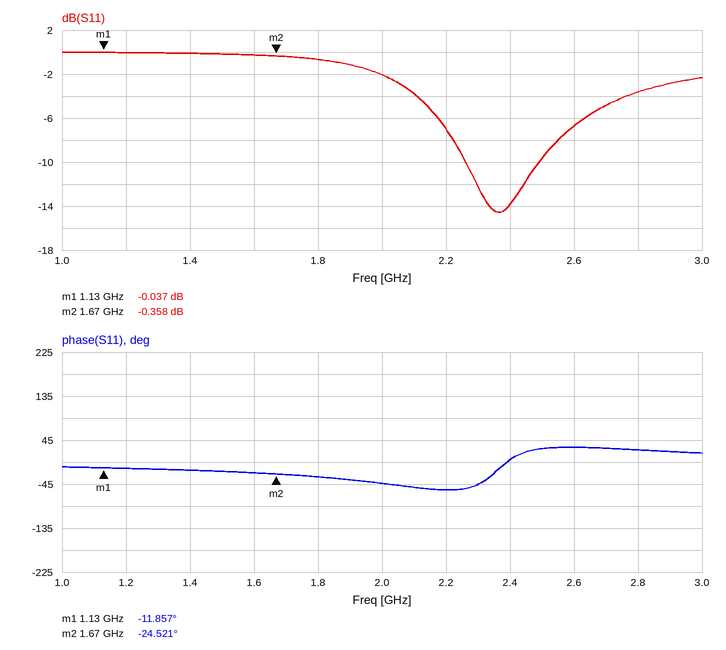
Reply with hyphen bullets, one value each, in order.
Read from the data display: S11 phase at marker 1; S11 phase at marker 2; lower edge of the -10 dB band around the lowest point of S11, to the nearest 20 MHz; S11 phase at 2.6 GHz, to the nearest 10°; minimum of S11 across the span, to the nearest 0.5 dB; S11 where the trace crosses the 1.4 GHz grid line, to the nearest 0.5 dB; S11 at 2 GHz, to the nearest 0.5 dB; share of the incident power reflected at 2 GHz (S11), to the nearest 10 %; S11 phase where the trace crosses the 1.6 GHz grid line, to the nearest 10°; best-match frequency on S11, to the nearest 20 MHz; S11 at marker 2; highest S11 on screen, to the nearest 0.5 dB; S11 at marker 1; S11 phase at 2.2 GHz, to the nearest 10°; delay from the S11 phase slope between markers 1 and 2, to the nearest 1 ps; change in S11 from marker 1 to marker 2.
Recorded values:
- -11.857°
- -24.521°
- 2.26 GHz
- 30°
- -14.5 dB
- 0.0 dB
- -2.0 dB
- 60 %
- -20°
- 2.36 GHz
- -0.358 dB
- 0.0 dB
- -0.037 dB
- -60°
- 65 ps
- -0.321 dB
